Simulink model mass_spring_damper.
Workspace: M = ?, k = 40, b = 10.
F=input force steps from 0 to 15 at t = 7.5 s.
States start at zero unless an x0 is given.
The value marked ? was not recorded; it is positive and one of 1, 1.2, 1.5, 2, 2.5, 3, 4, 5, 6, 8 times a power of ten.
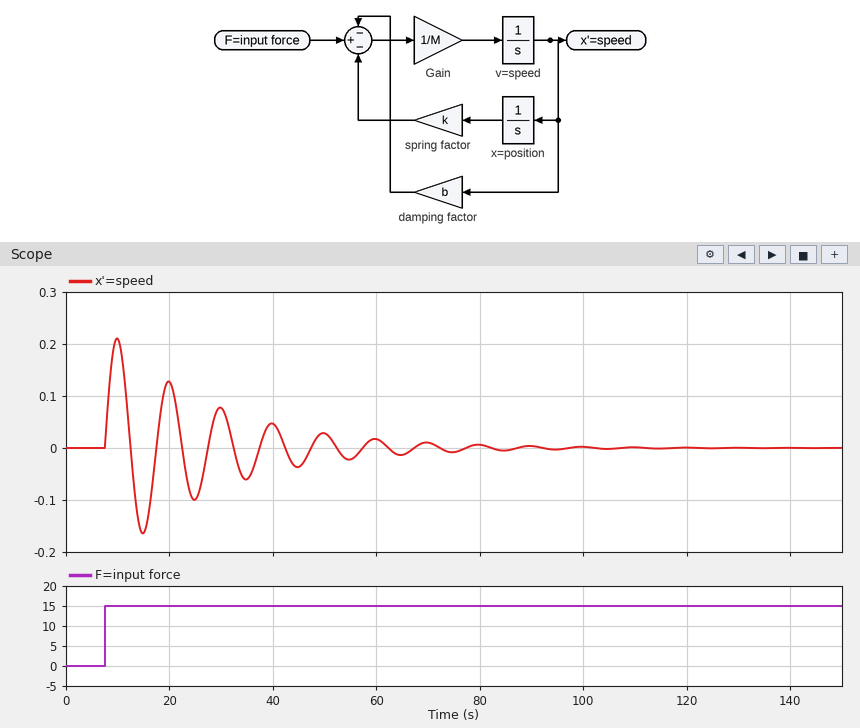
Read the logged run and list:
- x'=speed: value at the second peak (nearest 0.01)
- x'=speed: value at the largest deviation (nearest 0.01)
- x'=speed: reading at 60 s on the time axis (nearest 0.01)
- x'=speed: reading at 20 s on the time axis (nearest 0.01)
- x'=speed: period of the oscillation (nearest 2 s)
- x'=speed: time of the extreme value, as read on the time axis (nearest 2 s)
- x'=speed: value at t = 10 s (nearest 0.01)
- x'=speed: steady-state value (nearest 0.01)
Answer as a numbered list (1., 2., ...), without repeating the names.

1. 0.13
2. 0.21
3. 0.02
4. 0.13
5. 10 s
6. 10 s
7. 0.21
8. 0.00
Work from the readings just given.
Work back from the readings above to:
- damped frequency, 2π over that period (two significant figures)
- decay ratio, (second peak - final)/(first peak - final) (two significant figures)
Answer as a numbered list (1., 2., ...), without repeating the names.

1. 0.63 rad/s
2. 0.62
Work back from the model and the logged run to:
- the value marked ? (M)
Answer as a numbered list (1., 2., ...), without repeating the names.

1. 100
